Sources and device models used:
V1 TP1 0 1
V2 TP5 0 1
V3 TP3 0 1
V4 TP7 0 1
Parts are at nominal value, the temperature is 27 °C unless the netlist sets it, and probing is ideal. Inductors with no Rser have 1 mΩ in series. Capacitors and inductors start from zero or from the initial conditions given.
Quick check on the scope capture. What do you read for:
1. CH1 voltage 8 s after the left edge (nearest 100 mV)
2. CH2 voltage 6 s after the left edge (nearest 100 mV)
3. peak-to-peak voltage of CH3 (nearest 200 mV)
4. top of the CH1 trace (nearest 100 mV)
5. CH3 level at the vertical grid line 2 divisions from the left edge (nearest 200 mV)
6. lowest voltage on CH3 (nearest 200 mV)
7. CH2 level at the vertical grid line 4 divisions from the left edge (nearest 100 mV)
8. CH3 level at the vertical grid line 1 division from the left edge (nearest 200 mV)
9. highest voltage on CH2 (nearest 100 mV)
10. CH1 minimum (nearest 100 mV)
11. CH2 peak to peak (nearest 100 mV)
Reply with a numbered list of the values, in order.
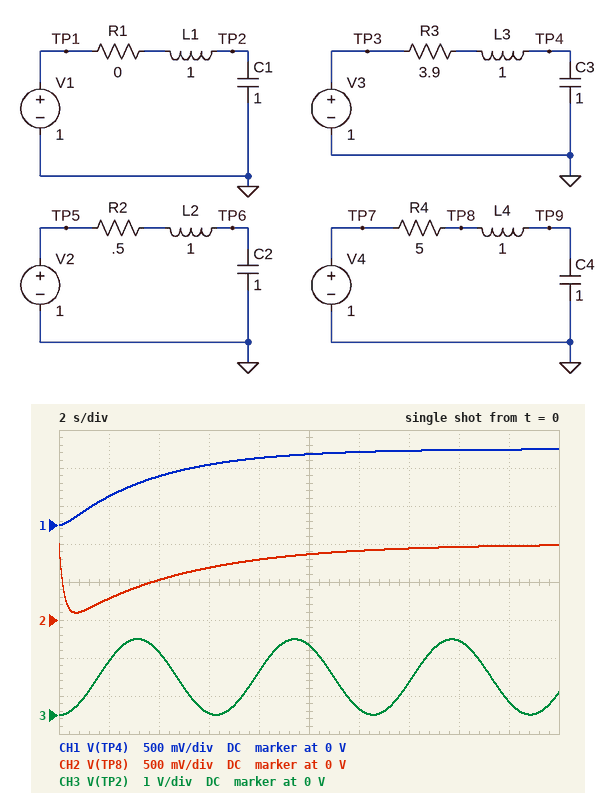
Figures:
1. 900 mV
2. 700 mV
3. 2.0 V
4. 1.0 V
5. 1.6 V
6. 0 V
7. 800 mV
8. 1.4 V
9. 1.0 V
10. 0 V
11. 900 mV
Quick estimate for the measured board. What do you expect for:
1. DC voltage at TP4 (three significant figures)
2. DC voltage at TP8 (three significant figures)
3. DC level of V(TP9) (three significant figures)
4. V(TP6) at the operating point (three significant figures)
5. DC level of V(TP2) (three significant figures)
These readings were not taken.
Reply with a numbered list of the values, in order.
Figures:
1. 1.00 V
2. 1.00 V
3. 1.00 V
4. 1.00 V
5. 1.00 V
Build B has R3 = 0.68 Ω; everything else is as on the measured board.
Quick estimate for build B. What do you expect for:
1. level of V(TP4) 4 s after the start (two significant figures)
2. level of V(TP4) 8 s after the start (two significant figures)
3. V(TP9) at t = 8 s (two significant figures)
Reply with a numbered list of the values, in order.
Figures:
1. 1.3 V
2. 960 mV
3. 800 mV
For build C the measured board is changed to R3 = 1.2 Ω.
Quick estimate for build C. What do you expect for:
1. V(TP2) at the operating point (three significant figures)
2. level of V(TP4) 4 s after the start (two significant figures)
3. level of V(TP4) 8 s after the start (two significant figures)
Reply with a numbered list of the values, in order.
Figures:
1. 1.00 V
2. 1.1 V
3. 990 mV
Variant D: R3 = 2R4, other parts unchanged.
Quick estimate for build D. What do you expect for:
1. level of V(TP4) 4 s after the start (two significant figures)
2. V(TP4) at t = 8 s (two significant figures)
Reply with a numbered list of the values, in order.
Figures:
1. 840 mV
2. 980 mV
